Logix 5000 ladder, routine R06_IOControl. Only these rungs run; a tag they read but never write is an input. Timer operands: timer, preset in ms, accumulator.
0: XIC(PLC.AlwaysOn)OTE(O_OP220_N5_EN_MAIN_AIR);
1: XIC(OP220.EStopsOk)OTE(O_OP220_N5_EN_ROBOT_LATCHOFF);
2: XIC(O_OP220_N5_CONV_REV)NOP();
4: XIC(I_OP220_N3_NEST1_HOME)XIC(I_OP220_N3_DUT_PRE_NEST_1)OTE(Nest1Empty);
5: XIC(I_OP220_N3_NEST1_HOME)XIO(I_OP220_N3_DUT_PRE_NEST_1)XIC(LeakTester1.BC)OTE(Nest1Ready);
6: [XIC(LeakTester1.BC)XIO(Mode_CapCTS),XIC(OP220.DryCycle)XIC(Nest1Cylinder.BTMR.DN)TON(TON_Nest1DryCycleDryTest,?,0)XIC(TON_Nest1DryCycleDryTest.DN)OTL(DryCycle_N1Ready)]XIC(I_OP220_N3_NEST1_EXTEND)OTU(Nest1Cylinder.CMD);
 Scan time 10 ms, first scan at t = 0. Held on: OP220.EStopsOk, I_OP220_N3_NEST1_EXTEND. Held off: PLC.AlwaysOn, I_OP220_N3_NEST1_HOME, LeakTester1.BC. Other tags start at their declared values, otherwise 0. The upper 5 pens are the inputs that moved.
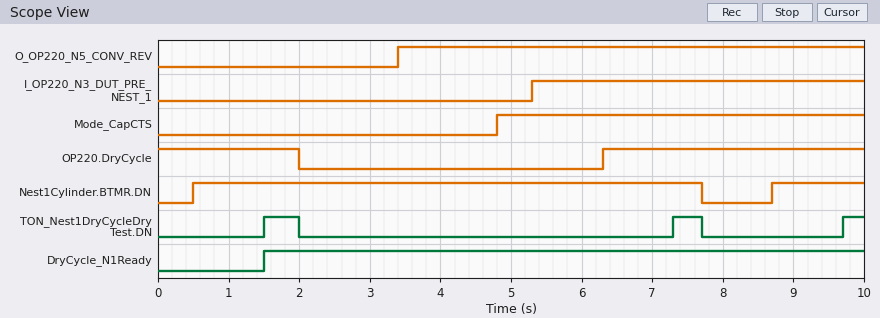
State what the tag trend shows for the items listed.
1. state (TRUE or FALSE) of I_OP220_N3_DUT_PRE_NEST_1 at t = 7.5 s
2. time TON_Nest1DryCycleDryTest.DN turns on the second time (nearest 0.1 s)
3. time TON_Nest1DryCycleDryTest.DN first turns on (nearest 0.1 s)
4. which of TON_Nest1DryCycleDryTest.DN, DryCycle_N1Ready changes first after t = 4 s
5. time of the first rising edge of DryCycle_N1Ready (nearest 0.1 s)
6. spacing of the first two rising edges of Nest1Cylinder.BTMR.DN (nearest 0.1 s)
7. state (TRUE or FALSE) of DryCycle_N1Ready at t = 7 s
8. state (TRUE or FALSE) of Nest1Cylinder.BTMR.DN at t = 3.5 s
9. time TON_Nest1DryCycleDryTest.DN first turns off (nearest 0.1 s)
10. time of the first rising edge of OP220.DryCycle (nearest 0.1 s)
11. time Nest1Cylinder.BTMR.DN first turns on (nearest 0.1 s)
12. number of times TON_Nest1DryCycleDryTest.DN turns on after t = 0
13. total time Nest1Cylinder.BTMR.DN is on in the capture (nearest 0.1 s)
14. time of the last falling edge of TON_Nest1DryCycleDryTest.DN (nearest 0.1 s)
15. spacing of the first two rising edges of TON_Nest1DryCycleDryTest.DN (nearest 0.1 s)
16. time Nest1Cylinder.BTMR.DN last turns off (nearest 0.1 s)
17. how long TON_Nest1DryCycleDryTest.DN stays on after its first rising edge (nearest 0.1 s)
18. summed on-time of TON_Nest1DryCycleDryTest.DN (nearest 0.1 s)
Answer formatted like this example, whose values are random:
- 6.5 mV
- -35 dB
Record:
- TRUE
- 7.3 s
- 1.5 s
- TON_Nest1DryCycleDryTest.DN
- 1.5 s
- 8.2 s
- TRUE
- TRUE
- 2.0 s
- 6.3 s
- 0.5 s
- 3
- 8.5 s
- 7.7 s
- 5.8 s
- 7.7 s
- 0.5 s
- 1.2 s
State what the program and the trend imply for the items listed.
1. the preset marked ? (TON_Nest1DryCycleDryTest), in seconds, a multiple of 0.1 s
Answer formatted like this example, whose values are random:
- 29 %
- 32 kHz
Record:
- 1.0 s
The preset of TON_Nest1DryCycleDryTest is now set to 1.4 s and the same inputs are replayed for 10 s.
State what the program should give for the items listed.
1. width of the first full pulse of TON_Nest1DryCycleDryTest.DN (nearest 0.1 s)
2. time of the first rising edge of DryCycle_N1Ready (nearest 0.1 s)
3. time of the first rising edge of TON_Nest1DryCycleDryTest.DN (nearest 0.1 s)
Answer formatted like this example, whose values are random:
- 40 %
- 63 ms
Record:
- 0.1 s
- 1.9 s
- 1.9 s
